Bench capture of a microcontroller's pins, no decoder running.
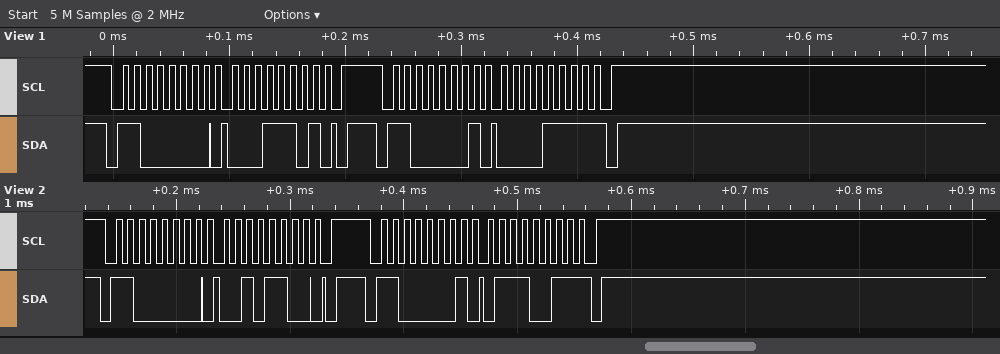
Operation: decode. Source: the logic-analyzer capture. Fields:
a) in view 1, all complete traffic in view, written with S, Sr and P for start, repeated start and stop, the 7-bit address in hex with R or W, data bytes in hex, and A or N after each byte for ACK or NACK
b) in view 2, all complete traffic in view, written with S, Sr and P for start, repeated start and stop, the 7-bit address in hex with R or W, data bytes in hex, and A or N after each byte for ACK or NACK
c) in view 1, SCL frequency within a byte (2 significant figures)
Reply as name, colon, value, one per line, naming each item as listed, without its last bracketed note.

in view 1, all complete traffic in view, written with S, Sr and P for start, repeated start and stop, the 7-bit address in hex with R or W, data bytes in hex, and A or N after each byte for ACK or NACK: S 60W A 1D A P S 60R A 0F N P
in view 2, all complete traffic in view, written with S, Sr and P for start, repeated start and stop, the 7-bit address in hex with R or W, data bytes in hex, and A or N after each byte for ACK or NACK: S 60W A 2C A P S 60R A 73 N P
in view 1, SCL frequency within a byte: 100 kHz
